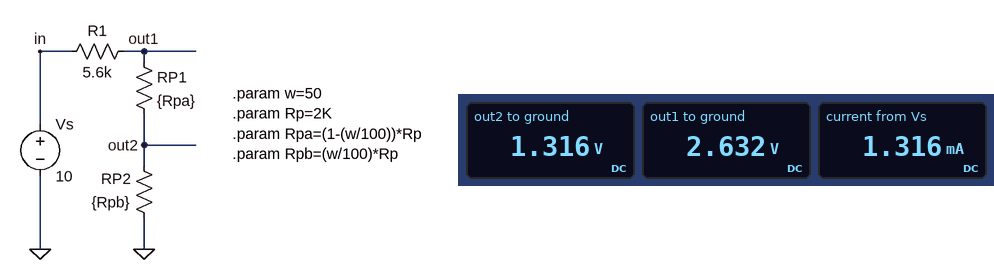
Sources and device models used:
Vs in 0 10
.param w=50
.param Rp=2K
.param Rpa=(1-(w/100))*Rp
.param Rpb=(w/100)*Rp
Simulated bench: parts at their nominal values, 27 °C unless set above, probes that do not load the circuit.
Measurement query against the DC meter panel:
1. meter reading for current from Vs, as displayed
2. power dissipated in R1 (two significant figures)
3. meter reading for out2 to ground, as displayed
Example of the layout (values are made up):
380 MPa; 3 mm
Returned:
1.316 mA; 9.7 mW; 1.316 V
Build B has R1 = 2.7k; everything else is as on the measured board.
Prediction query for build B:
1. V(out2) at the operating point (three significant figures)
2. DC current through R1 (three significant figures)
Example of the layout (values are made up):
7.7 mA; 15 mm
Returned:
2.13 V; 2.13 mA
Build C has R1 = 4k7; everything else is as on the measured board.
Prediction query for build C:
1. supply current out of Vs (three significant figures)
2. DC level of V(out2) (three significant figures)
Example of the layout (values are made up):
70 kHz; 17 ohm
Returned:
1.49 mA; 1.49 V
